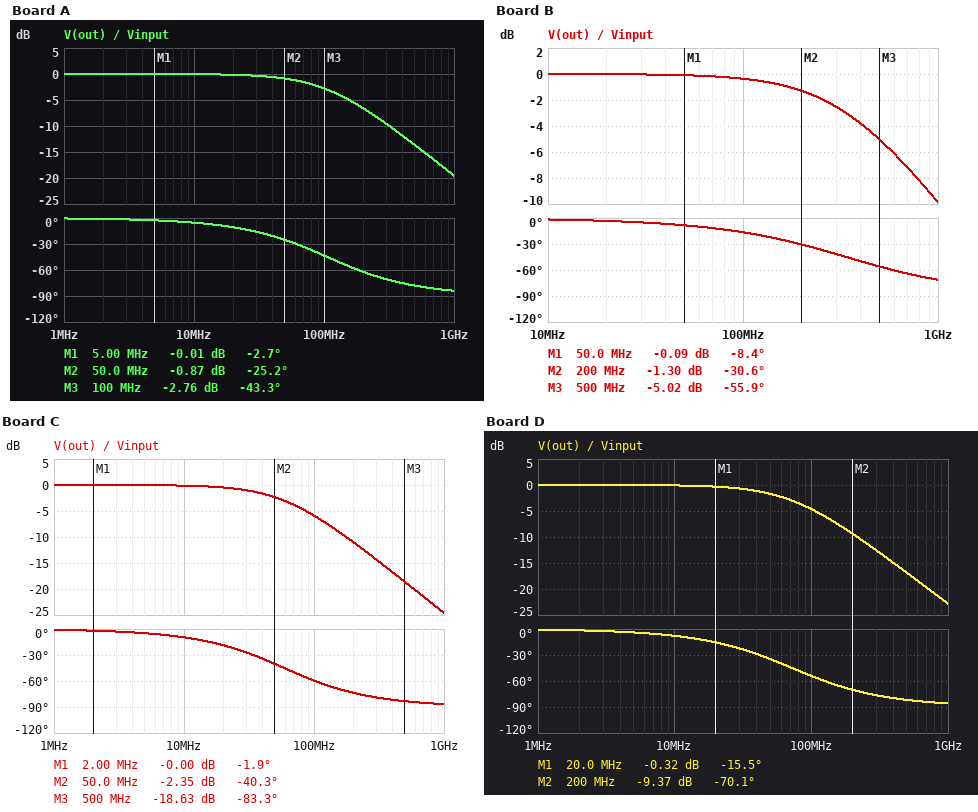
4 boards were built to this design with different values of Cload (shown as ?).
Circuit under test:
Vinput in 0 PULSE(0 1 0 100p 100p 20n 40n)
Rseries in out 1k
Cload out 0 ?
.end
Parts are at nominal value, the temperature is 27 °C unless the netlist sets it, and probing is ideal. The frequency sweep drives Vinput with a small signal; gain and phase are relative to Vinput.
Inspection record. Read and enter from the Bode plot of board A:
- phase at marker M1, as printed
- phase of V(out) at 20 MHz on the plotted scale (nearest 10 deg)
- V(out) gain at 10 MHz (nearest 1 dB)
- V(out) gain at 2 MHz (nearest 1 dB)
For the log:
-2.7 deg
-10 deg
0 dB
0 dB
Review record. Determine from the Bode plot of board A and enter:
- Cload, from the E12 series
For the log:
1.5 pF
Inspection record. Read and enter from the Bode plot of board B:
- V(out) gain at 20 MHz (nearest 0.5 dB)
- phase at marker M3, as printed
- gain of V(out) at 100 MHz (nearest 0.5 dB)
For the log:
0 dB
-55.9 deg
-0.5 dB
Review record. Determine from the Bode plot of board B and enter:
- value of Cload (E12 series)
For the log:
470 fF
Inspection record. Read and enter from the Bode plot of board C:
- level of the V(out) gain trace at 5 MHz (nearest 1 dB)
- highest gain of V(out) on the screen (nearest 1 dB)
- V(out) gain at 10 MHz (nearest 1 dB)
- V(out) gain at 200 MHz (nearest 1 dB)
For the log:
0 dB
0 dB
0 dB
-11 dB
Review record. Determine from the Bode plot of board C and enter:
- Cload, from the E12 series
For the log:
2.7 pF
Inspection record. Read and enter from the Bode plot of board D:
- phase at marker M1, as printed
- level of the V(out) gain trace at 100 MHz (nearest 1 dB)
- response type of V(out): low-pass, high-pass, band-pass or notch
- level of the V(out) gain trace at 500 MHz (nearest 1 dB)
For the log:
-15.5 deg
-5 dB
low-pass
-17 dB
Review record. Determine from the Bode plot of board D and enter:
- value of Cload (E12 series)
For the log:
2.2 pF
